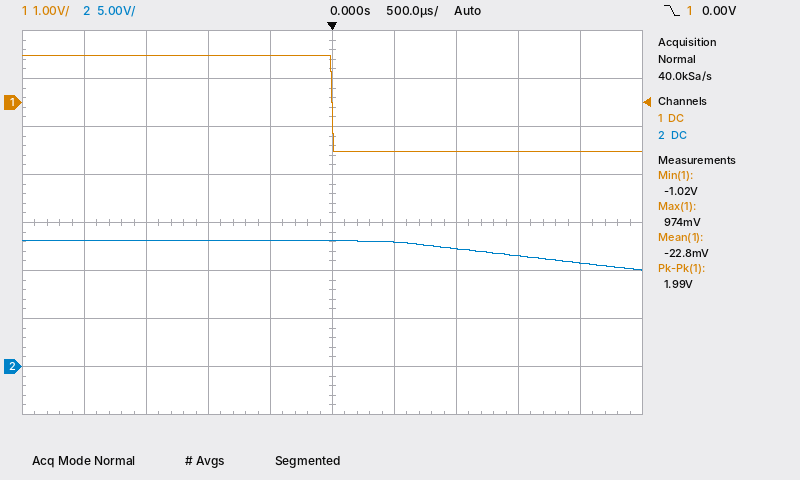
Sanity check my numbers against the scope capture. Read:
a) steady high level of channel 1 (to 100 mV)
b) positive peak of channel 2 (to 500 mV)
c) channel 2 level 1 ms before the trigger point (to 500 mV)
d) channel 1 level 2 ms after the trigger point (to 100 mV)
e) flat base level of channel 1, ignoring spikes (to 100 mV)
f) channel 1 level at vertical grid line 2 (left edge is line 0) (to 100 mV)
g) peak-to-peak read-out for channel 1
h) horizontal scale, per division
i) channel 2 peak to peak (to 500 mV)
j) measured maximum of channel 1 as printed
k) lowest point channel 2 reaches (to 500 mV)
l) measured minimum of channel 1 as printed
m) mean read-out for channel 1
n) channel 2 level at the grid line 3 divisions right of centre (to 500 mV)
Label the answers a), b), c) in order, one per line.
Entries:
a) 1.0 V
b) 13.0 V
c) 13.0 V
d) -1.0 V
e) -1.0 V
f) 1.0 V
g) 1.99 V
h) 500 µs
i) 3.0 V
j) 974 mV
k) 10.0 V
l) -1.02 V
m) -22.8 mV
n) 11.5 V
